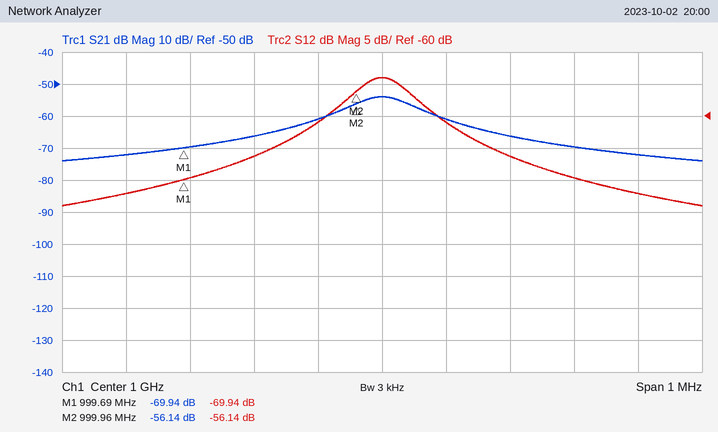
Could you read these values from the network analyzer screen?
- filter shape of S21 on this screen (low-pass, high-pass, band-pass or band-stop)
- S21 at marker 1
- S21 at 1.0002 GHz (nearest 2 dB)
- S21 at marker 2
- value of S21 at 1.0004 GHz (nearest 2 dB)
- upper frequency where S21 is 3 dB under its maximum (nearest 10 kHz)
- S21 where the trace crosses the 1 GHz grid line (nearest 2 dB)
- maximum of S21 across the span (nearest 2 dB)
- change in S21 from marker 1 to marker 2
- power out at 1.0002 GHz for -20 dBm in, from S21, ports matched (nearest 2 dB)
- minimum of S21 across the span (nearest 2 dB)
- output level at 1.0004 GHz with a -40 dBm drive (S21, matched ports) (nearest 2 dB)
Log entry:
band-pass
-69.94 dB
-66 dB
-56.14 dB
-72 dB
1.00005 GHz
-54 dB
-54 dB
13.80 dB
-86 dBm
-74 dB
-112 dBm
